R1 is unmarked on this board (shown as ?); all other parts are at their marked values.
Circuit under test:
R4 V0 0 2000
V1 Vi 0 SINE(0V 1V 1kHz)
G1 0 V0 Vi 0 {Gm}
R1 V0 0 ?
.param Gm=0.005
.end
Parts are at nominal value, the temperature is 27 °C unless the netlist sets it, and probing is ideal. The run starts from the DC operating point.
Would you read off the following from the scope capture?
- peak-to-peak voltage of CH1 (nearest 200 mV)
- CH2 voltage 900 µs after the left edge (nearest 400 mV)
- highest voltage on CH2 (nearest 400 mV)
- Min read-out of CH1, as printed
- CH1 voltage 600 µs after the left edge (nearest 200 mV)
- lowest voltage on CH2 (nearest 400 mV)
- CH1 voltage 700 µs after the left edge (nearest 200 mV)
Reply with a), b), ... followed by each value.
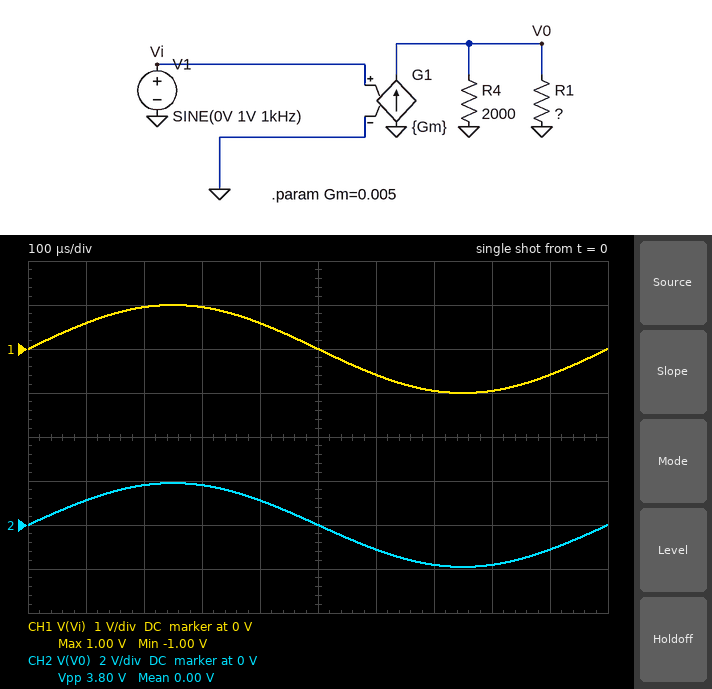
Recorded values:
a) 2.0 V
b) -1.2 V
c) 2.0 V
d) -1.00 V
e) -600 mV
f) -2.0 V
g) -1.0 V
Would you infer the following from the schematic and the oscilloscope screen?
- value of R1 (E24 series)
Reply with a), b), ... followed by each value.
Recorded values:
a) 470 Ω
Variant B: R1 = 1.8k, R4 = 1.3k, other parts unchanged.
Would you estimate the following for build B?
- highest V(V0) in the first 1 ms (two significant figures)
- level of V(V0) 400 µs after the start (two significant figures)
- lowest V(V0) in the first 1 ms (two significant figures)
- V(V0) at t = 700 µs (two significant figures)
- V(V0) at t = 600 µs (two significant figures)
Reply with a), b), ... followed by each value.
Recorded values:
a) 3.8 V
b) 2.2 V
c) -3.8 V
d) -3.6 V
e) -2.2 V
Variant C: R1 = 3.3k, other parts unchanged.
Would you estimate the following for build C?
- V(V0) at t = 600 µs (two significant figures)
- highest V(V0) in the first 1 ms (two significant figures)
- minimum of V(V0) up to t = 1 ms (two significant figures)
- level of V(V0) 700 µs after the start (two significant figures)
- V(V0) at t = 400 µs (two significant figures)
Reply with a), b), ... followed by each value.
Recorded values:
a) -3.7 V
b) 6.2 V
c) -6.2 V
d) -5.9 V
e) 3.7 V
